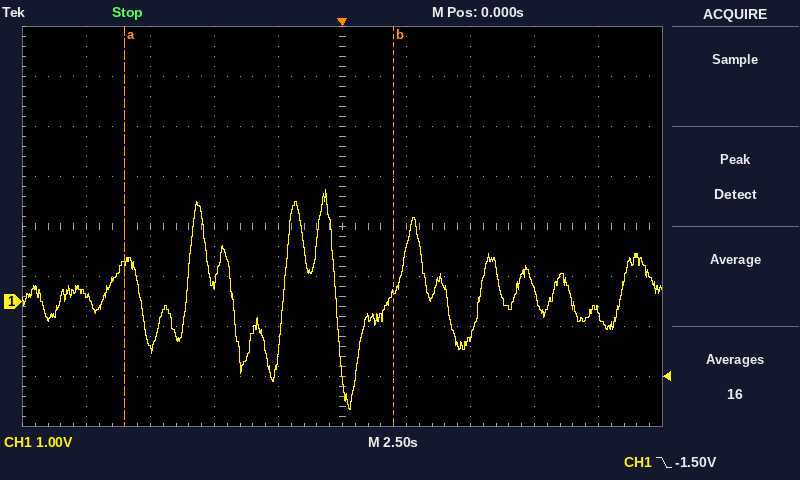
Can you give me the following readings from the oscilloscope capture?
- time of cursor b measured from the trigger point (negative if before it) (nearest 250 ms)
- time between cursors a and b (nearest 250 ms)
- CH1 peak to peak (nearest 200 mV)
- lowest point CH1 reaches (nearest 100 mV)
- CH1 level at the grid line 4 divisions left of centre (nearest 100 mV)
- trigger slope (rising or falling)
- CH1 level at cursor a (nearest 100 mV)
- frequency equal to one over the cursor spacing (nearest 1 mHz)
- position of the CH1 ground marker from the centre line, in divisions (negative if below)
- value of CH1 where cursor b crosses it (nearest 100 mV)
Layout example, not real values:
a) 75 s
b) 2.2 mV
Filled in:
a) +2.00 s
b) 10.50 s
c) 4.4 V
d) -2.2 V
e) 200 mV
f) falling
g) 800 mV
h) 95 mHz
i) -1.5 div
j) 200 mV
